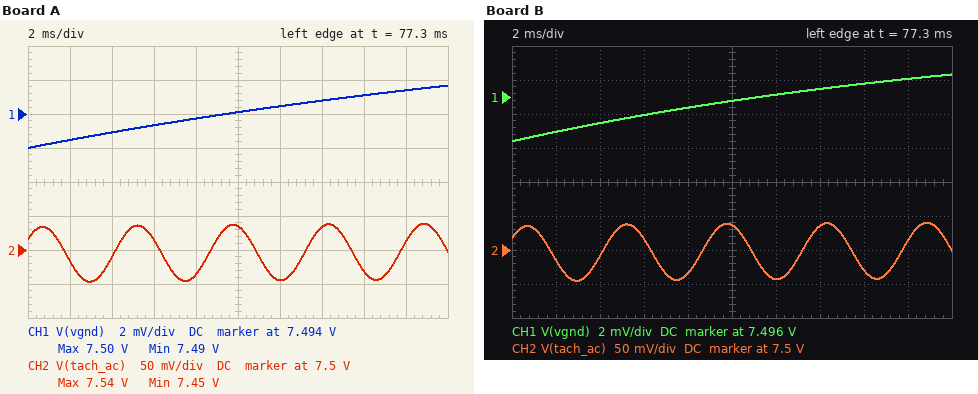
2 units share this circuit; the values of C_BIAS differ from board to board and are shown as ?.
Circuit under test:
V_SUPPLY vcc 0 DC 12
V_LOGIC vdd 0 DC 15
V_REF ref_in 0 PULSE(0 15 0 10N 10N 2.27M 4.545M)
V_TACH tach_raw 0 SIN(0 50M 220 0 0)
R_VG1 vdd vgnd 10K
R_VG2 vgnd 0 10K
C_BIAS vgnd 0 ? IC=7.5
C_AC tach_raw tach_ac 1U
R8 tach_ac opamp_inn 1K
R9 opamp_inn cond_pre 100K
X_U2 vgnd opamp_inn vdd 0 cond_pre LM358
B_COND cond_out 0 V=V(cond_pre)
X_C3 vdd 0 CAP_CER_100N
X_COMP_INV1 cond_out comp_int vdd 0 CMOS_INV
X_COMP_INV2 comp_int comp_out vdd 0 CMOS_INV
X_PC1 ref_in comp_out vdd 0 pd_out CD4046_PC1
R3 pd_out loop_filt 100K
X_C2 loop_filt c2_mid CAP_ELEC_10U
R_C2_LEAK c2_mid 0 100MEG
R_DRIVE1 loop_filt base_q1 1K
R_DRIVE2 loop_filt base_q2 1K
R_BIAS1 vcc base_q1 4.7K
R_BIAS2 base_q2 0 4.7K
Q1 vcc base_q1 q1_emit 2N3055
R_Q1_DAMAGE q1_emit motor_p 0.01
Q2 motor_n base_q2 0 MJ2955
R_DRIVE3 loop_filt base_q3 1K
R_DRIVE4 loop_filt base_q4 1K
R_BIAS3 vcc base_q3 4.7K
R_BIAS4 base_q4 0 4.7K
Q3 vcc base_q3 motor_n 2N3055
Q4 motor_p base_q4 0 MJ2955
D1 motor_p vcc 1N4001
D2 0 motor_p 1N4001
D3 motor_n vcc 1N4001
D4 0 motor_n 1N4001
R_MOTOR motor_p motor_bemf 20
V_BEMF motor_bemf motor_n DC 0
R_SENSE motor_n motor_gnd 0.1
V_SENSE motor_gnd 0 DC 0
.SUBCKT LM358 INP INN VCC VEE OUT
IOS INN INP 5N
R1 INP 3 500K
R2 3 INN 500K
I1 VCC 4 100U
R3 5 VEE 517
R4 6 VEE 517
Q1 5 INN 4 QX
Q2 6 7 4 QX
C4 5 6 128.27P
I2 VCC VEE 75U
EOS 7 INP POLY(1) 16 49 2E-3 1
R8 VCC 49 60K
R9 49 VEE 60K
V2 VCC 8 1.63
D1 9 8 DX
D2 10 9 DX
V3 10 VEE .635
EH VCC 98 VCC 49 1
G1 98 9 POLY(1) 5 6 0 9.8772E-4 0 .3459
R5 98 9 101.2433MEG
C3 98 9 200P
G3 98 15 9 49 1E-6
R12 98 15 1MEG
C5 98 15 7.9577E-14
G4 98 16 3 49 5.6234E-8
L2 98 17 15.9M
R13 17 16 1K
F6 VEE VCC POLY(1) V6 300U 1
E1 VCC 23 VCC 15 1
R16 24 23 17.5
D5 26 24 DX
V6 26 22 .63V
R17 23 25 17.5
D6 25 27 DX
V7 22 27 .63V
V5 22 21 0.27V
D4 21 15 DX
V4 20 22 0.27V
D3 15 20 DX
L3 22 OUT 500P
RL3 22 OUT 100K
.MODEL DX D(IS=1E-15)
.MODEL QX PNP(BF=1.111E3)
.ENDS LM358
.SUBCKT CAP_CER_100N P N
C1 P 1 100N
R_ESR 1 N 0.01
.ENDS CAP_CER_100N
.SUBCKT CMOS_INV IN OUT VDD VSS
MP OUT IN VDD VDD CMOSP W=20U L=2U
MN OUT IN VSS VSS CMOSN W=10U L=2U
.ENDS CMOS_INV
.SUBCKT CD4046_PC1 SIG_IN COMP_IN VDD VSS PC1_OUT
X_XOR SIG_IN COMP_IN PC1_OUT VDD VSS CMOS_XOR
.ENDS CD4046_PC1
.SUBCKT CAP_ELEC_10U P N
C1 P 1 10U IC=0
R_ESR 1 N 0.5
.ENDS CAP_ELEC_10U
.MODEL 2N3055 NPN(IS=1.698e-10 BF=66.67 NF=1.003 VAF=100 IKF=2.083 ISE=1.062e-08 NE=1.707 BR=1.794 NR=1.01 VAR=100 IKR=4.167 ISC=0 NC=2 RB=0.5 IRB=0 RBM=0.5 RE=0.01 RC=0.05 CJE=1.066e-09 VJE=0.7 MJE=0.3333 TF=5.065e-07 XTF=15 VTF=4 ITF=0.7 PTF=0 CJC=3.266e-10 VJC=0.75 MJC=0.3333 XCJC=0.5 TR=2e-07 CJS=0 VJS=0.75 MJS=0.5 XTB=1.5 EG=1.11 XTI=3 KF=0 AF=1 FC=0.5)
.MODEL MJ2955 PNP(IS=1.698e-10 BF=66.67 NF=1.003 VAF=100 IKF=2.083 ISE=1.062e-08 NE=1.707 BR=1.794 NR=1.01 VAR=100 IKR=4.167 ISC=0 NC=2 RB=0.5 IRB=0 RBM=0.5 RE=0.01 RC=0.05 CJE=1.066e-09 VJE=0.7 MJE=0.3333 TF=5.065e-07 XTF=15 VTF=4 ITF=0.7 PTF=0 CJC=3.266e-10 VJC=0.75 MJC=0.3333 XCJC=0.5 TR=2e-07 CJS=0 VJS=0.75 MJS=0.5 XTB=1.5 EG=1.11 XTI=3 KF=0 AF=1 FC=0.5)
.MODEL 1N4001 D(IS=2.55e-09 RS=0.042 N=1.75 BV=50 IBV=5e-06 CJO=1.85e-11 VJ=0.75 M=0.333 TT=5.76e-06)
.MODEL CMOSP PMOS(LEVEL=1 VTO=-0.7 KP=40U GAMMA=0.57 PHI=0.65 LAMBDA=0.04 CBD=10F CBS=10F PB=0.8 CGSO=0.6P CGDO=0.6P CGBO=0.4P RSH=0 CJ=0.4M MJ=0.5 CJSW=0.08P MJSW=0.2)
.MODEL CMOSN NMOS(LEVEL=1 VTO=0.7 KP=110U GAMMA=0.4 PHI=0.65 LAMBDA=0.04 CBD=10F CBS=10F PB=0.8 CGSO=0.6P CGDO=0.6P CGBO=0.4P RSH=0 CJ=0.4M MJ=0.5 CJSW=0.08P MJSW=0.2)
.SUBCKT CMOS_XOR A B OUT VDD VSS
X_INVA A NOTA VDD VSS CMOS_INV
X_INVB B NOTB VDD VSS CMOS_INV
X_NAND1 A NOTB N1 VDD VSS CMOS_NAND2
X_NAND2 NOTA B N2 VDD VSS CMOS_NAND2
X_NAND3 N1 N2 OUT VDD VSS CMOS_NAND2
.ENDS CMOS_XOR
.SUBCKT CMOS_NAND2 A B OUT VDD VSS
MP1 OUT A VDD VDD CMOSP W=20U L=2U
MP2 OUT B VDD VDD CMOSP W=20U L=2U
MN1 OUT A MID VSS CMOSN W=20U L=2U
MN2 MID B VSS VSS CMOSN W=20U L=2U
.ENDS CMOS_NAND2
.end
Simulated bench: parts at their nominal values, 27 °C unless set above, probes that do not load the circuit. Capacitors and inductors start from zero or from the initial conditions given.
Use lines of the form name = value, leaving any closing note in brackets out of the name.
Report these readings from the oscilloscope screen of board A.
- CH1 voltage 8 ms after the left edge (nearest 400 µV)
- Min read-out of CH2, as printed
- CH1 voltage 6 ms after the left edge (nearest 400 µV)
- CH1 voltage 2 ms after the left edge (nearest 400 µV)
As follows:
CH1 voltage 8 ms after the left edge = 7.4936 V
Min read-out of CH2, as printed = 7.45 V
CH1 voltage 6 ms after the left edge = 7.4932 V
CH1 voltage 2 ms after the left edge = 7.4924 V
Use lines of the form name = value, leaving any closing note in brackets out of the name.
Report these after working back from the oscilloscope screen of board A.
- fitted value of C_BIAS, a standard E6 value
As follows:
fitted value of C_BIAS, a standard E6 value = 6.8 µF
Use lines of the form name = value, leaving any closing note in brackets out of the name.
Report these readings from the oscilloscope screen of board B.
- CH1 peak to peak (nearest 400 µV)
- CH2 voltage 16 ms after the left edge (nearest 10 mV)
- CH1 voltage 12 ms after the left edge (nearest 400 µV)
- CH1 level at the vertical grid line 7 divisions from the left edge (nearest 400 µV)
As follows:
CH1 peak to peak = 4.0 mV
CH2 voltage 16 ms after the left edge = 7.47 V
CH1 voltage 12 ms after the left edge = 7.4960 V
CH1 level at the vertical grid line 7 divisions from the left edge = 7.4964 V
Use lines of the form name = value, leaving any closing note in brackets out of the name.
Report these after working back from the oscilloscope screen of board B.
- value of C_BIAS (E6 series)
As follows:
value of C_BIAS = 4.7 µF
